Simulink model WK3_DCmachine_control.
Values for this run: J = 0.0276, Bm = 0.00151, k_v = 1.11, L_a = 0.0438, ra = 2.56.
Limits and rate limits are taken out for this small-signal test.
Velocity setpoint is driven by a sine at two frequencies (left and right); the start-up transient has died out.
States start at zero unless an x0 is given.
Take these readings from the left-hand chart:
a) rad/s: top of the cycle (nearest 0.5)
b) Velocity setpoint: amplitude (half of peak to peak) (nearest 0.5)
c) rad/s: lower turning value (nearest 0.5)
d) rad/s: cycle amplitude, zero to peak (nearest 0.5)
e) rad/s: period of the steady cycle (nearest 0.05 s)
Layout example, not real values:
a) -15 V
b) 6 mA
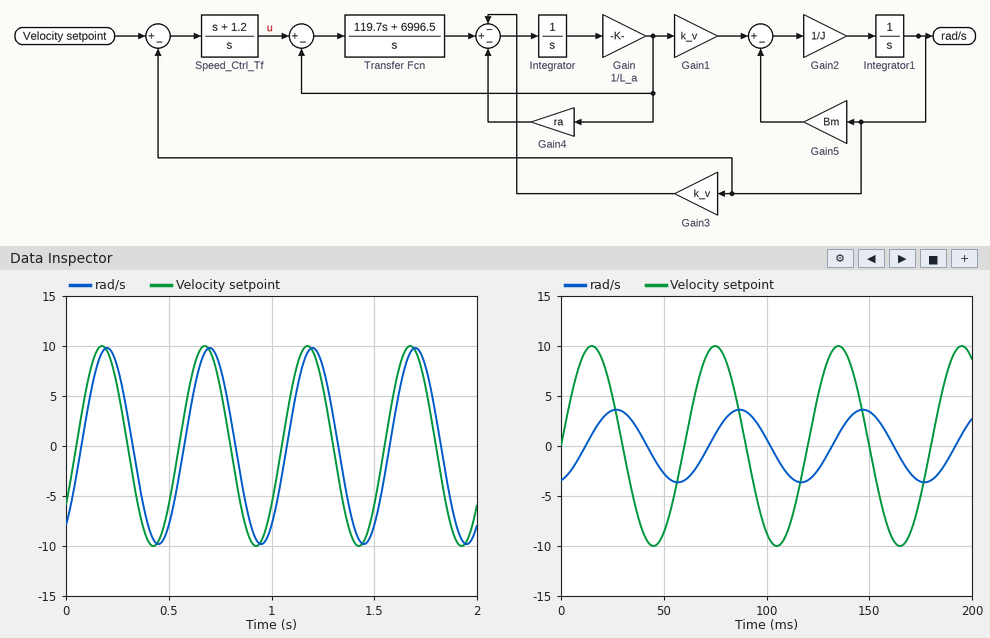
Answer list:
a) 10.0
b) 10.0
c) -10.0
d) 10.0
e) 0.50 s
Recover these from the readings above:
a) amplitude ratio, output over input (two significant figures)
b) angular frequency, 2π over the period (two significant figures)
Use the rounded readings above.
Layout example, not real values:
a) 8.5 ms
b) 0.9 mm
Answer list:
a) 1.0
b) 13 rad/s
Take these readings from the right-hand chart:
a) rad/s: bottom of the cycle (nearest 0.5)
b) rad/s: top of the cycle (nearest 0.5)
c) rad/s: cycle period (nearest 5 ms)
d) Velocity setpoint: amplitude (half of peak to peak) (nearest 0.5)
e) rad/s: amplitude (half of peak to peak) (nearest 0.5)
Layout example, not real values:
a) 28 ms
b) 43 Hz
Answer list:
a) -3.5
b) 3.5
c) 60 ms
d) 10.0
e) 3.5
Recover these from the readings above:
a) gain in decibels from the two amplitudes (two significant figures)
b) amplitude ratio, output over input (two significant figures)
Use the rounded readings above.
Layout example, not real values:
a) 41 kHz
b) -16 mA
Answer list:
a) -9.1 dB
b) 0.35
